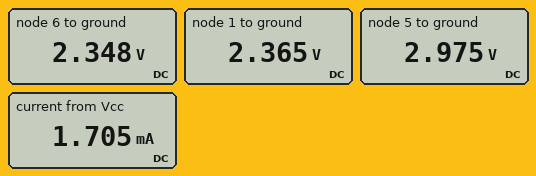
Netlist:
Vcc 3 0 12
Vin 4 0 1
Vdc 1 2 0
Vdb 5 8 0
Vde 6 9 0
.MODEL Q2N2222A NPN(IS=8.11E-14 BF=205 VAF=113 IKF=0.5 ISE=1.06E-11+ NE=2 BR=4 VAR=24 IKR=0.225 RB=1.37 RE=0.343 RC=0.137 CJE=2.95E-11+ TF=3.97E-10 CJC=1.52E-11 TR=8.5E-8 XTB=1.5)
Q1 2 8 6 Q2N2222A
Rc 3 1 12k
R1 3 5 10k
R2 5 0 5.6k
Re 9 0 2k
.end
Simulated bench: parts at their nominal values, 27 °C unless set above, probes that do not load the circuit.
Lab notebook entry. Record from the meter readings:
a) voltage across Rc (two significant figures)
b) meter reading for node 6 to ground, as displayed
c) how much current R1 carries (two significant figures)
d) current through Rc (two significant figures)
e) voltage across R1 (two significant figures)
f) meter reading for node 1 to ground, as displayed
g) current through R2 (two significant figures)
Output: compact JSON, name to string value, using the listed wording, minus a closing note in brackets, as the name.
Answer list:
{"voltage across Rc": "9.6 V", "meter reading for node 6 to ground, as displayed": "2.348 V", "how much current R1 carries": "900 µA", "current through Rc": "800 µA", "voltage across R1": "9.0 V", "meter reading for node 1 to ground, as displayed": "2.365 V", "current through R2": "530 µA"}
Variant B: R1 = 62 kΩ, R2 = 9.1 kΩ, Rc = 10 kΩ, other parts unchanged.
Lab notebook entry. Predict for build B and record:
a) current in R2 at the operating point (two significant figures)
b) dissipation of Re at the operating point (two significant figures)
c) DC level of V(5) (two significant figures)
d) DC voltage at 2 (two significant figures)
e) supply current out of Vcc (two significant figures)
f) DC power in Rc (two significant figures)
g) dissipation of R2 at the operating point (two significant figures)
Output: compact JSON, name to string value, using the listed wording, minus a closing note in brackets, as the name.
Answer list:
{"current in R2 at the operating point": "170 µA", "dissipation of Re at the operating point": "430 µW", "DC level of V(5)": "1.5 V", "DC voltage at 2": "7.4 V", "supply current out of Vcc": "630 µA", "DC power in Rc": "2.1 mW", "dissipation of R2 at the operating point": "250 µW"}
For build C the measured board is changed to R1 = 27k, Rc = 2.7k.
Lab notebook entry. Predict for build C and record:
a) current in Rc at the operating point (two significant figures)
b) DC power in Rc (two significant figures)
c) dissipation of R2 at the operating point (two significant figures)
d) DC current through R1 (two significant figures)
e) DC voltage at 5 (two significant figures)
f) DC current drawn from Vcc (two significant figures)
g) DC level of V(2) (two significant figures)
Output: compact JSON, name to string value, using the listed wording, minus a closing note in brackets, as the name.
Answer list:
{"current in Rc at the operating point": "720 µA", "DC power in Rc": "1.4 mW", "dissipation of R2 at the operating point": "740 µW", "DC current through R1": "370 µA", "DC voltage at 5": "2.0 V", "DC current drawn from Vcc": "1.1 mA", "DC level of V(2)": "10 V"}
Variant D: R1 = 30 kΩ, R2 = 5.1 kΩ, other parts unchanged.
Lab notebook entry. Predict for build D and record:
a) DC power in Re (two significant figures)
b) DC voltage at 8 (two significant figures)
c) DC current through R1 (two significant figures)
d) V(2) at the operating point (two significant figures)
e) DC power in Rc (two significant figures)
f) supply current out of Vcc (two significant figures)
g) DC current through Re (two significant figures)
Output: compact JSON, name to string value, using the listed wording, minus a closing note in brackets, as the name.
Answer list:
{"DC power in Re": "650 µW", "DC voltage at 8": "1.7 V", "DC current through R1": "340 µA", "V(2) at the operating point": "5.2 V", "DC power in Rc": "3.9 mW", "supply current out of Vcc": "910 µA", "DC current through Re": "570 µA"}
